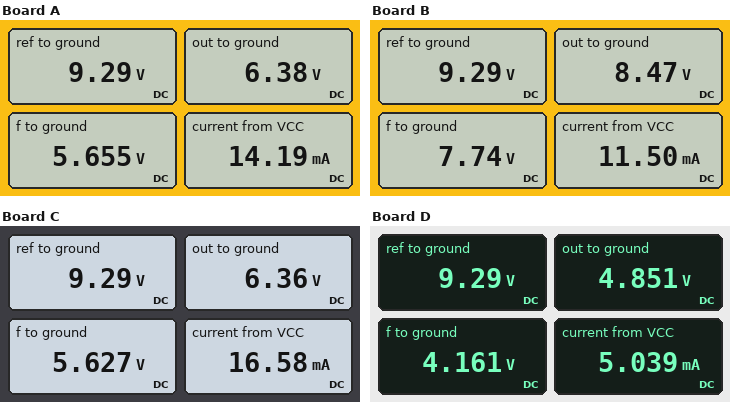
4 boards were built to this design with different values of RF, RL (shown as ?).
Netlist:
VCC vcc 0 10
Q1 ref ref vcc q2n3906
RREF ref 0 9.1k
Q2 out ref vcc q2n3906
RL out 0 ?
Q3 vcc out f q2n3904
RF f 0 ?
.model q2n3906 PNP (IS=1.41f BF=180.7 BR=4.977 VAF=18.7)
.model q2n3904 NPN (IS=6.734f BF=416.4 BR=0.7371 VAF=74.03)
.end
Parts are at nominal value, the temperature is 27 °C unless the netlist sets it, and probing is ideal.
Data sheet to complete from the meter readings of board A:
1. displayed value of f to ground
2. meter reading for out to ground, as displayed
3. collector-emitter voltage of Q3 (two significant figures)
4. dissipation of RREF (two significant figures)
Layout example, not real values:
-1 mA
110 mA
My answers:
5.655 V
6.38 V
4.3 V
9.5 mW
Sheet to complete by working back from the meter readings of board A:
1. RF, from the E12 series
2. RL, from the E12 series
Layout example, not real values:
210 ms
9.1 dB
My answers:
470 Ω
5.6 kΩ
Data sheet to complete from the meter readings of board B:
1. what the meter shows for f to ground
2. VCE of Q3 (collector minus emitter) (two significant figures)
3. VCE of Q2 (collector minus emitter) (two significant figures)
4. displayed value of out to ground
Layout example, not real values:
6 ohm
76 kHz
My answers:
7.74 V
2.3 V
-1.5 V
8.47 V
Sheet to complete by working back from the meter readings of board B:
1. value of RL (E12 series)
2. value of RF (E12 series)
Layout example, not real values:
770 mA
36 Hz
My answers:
8.2 kΩ
820 Ω
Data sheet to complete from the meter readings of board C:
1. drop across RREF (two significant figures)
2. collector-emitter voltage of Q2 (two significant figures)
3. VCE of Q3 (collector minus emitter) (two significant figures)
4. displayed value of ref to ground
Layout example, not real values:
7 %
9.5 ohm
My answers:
9.3 V
-3.6 V
4.4 V
9.29 V
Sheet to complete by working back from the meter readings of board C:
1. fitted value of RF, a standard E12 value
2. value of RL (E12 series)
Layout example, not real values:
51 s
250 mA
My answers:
390 Ω
5.6 kΩ
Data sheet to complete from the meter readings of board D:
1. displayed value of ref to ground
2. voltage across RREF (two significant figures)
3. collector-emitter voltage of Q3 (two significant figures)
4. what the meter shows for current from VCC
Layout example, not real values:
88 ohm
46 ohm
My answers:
9.29 V
9.3 V
5.8 V
5.039 mA
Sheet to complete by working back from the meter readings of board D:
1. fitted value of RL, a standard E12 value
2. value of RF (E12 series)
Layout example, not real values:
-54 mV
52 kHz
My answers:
3.9 kΩ
1.5 kΩ
